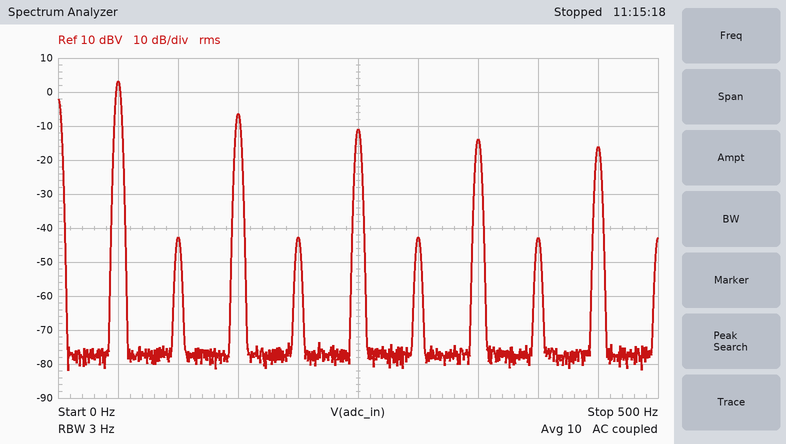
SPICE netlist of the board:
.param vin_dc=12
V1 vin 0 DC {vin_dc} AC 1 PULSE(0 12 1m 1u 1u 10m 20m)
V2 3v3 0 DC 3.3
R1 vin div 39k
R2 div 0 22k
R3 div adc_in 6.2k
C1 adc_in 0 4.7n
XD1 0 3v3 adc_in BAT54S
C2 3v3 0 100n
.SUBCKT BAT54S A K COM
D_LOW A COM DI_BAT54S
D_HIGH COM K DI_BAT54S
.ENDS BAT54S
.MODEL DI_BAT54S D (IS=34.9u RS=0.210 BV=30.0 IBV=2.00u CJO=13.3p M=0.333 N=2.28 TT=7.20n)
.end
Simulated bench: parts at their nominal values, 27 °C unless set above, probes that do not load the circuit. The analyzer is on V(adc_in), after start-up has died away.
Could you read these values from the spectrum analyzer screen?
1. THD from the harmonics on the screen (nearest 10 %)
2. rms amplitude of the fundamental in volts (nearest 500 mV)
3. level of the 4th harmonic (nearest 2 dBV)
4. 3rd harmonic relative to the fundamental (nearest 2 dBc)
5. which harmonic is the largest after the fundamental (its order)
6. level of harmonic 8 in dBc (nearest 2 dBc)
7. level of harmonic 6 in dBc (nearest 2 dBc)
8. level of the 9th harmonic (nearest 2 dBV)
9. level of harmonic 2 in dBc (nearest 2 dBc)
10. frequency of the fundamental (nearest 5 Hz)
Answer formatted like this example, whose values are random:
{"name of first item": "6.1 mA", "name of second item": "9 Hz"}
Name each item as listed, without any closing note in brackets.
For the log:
{"THD from the harmonics on the screen": "40 %", "rms amplitude of the fundamental in volts": "1.5 V", "level of the 4th harmonic": "-42 dBV", "3rd harmonic relative to the fundamental": "-10 dBc", "which harmonic is the largest after the fundamental": "3", "level of harmonic 8 in dBc": "-46 dBc", "level of harmonic 6 in dBc": "-46 dBc", "level of the 9th harmonic": "-16 dBV", "level of harmonic 2 in dBc": "-46 dBc", "frequency of the fundamental": "50 Hz"}
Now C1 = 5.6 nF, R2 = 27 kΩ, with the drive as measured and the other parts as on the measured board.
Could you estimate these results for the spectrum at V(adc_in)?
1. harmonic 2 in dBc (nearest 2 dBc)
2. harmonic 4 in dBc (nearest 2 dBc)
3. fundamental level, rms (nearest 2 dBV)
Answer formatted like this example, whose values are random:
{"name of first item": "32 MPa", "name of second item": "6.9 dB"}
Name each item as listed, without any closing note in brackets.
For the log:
{"harmonic 2 in dBc": "-42 dBc", "harmonic 4 in dBc": "-42 dBc", "fundamental level, rms": "4 dBV"}
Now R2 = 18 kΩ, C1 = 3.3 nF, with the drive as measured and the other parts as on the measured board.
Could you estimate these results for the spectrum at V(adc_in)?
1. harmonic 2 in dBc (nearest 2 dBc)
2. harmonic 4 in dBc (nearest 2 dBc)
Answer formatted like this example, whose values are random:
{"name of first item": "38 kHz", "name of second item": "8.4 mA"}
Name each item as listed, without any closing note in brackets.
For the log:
{"harmonic 2 in dBc": "-54 dBc", "harmonic 4 in dBc": "-54 dBc"}
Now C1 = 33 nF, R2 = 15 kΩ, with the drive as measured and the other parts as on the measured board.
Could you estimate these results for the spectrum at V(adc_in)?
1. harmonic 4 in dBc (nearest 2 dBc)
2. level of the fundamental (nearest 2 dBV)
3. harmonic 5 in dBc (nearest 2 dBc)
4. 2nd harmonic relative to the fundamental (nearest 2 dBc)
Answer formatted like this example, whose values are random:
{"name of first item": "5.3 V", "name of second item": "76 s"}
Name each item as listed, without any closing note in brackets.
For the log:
{"harmonic 4 in dBc": "-58 dBc", "level of the fundamental": "2 dBV", "harmonic 5 in dBc": "-16 dBc", "2nd harmonic relative to the fundamental": "-56 dBc"}
